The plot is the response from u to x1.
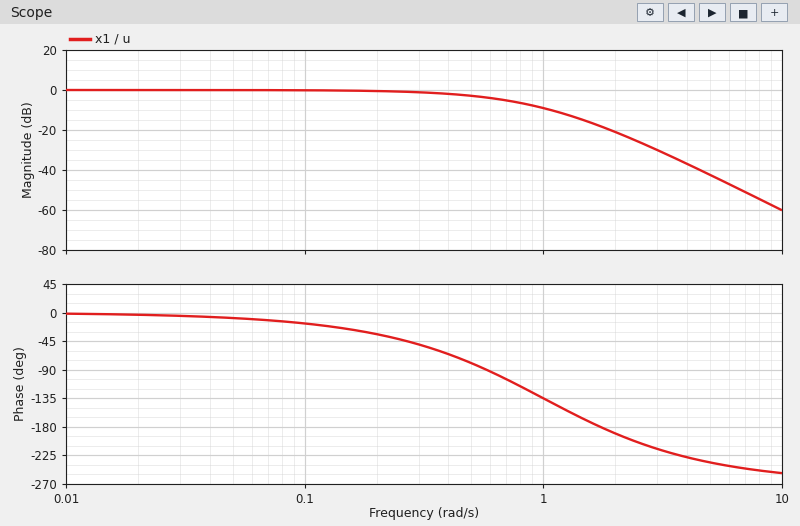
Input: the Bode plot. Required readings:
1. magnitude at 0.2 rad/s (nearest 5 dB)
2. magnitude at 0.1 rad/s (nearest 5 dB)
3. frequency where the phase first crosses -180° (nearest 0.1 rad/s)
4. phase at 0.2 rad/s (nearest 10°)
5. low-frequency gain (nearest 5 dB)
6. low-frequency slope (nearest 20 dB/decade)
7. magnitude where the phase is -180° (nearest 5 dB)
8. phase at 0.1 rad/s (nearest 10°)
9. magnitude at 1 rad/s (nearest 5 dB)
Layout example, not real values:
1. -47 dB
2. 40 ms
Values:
1. 0 dB
2. 0 dB
3. 1.7 rad/s
4. -30°
5. 0 dB
6. 0 dB/decade
7. -20 dB
8. -20°
9. -10 dB
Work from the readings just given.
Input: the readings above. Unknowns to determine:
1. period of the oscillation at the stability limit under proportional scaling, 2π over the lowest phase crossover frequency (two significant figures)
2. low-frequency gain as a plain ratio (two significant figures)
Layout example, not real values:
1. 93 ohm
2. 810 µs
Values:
1. 3.7 s
2. 1.0
